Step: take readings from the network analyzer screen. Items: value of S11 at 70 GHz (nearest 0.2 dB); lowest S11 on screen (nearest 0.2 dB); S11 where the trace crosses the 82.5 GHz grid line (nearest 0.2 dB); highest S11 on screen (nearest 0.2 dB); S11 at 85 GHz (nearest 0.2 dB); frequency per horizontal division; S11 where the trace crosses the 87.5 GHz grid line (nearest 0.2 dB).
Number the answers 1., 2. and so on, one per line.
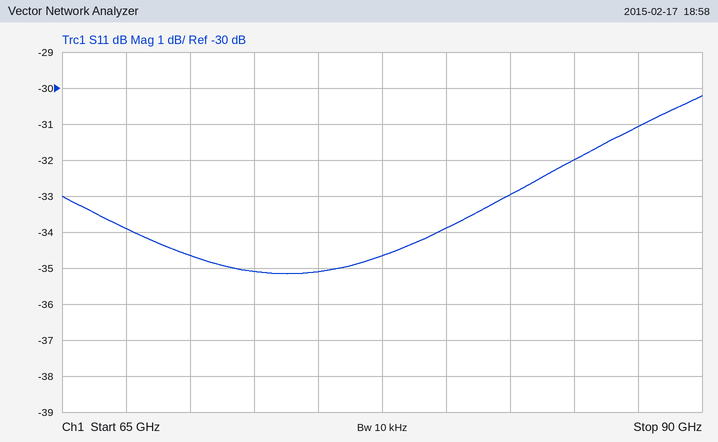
1. -34.6 dB
2. -35.2 dB
3. -33.0 dB
4. -30.2 dB
5. -32.0 dB
6. 2.5 GHz
7. -31.0 dB
